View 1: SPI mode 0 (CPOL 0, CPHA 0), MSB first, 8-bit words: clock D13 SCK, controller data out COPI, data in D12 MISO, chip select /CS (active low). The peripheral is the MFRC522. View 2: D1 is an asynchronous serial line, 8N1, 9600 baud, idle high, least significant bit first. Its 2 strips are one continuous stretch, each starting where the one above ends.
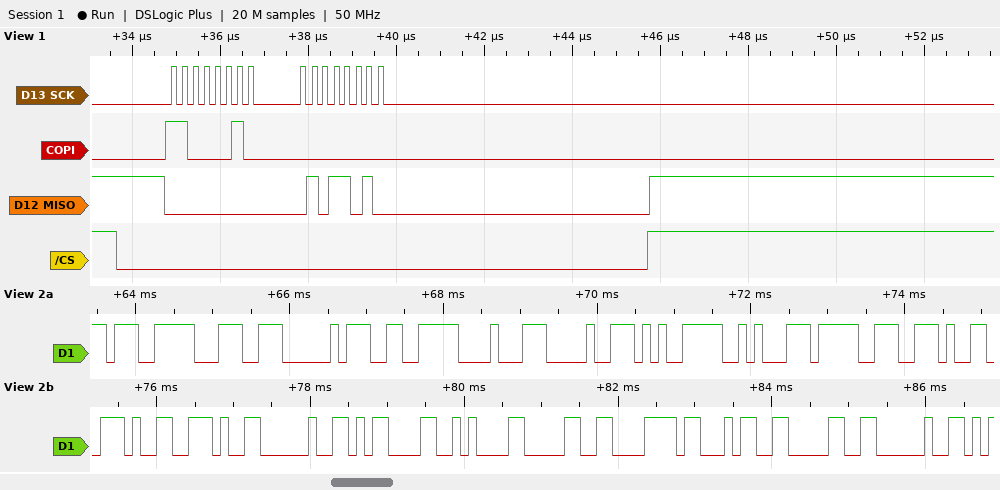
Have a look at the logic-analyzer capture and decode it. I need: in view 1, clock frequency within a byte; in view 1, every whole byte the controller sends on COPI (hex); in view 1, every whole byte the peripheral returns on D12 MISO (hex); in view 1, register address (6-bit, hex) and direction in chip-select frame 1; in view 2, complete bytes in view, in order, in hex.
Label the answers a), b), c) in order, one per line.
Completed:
a) 4 MHz
b) 0xC2 0x00
c) 0x00 0x5A
d) 0x21 read
e) E7 9C A0 E6 88 90 E5 8A 9F 2E 2E 2E 20 0D 0A 30 78 34 30 20
